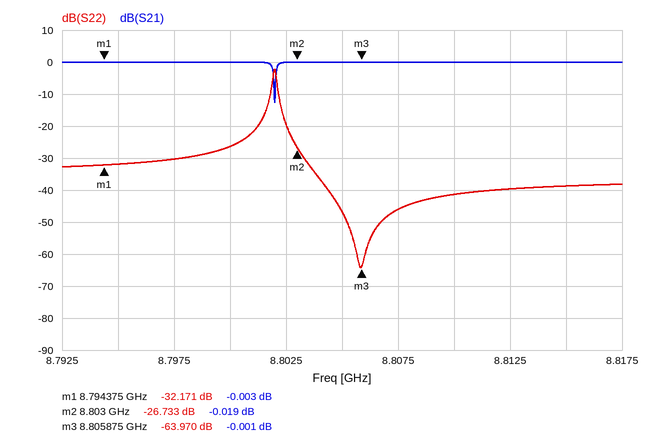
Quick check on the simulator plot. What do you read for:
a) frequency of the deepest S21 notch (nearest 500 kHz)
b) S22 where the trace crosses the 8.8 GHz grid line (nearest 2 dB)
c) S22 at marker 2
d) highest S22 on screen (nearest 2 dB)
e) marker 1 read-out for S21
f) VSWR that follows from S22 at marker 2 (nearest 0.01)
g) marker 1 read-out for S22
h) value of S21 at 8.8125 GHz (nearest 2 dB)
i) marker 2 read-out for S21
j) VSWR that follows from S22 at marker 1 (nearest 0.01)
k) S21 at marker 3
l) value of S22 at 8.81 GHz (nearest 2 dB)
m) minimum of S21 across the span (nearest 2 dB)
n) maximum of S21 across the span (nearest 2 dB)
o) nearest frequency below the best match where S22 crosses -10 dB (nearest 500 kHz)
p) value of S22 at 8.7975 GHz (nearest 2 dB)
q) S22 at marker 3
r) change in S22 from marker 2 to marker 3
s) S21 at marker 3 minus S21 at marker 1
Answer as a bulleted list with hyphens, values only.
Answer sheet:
- 8.8020 GHz
- -26 dB
- -26.733 dB
- -2 dB
- -0.003 dB
- 1.10
- -32.171 dB
- 0 dB
- -0.019 dB
- 1.05
- -0.001 dB
- -42 dB
- -12 dB
- 0 dB
- 8.8020 GHz
- -30 dB
- -63.970 dB
- -37.237 dB
- 0.002 dB
